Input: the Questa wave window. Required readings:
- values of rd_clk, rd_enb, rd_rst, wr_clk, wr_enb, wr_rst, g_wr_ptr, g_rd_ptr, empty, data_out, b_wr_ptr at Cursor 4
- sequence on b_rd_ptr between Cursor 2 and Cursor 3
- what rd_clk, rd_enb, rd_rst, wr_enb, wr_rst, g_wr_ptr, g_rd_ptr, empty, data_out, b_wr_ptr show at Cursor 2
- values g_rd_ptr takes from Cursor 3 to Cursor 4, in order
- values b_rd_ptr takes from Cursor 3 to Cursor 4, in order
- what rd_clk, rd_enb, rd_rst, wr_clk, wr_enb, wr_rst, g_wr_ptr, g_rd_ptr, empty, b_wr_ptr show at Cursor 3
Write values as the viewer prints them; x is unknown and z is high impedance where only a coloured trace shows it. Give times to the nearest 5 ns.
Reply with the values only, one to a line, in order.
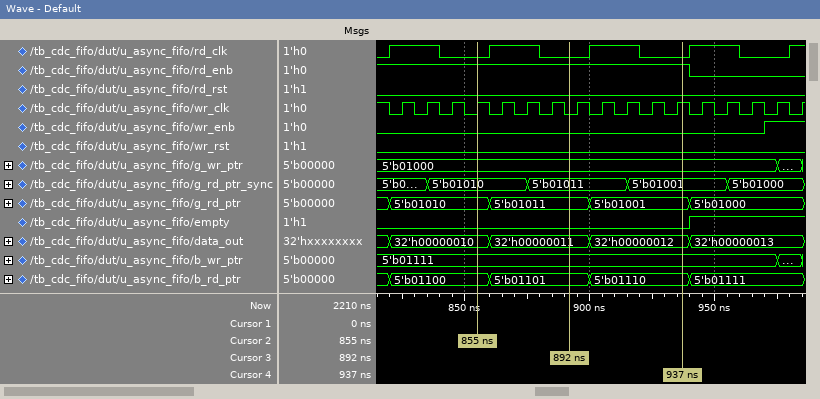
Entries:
rd_clk=0, rd_enb=1, rd_rst=0, wr_clk=1, wr_enb=0, wr_rst=0, g_wr_ptr=5'b01000, g_rd_ptr=5'b01001, empty=0, data_out=32'h00000012, b_wr_ptr=5'b01111
5'b01100, 5'b01101
rd_clk=0, rd_enb=1, rd_rst=0, wr_enb=0, wr_rst=0, g_wr_ptr=5'b01000, g_rd_ptr=5'b01010, empty=0, data_out=32'h00000010, b_wr_ptr=5'b01111
5'b01011, 5'b01001
5'b01101, 5'b01110
rd_clk=0, rd_enb=1, rd_rst=0, wr_clk=0, wr_enb=0, wr_rst=0, g_wr_ptr=5'b01000, g_rd_ptr=5'b01011, empty=0, b_wr_ptr=5'b01111
